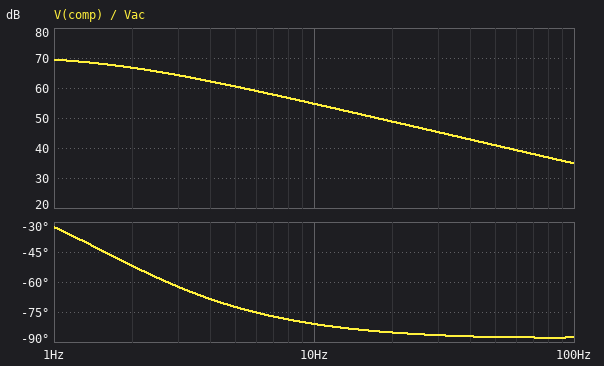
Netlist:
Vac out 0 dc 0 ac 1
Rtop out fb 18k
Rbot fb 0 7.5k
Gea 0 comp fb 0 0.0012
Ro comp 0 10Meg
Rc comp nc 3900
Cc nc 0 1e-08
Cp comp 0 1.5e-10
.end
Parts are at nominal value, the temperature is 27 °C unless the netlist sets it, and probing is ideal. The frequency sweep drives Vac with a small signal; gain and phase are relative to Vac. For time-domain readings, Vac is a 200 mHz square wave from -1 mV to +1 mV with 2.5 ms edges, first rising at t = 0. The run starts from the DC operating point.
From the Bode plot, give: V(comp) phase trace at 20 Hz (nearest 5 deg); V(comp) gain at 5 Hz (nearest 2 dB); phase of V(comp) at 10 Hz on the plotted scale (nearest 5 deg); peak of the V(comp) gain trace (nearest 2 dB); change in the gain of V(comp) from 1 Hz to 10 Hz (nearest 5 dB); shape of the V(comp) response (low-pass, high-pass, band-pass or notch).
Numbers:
-85 deg
60 dB
-80 deg
70 dB
-15 dB
low-pass
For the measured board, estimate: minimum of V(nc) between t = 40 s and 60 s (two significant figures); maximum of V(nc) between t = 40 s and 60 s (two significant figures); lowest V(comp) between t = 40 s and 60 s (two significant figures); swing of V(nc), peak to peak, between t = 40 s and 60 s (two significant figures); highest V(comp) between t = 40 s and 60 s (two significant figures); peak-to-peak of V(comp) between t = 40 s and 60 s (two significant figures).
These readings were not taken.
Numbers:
-3.5 V
3.5 V
-3.5 V
7.1 V
3.5 V
7.1 V
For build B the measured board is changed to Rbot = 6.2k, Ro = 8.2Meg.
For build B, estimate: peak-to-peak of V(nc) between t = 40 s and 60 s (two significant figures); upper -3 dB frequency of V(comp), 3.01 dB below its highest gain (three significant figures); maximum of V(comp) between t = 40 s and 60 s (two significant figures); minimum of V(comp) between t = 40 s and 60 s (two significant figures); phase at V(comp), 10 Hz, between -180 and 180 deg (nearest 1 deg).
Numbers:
5.0 V
1.91 Hz
2.5 V
-2.5 V
-79 deg
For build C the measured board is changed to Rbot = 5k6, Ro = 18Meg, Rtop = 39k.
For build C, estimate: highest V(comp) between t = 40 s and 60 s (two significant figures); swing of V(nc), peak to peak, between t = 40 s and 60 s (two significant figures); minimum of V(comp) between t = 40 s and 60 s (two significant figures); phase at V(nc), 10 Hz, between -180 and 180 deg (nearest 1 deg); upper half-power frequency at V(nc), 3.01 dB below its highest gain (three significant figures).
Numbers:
2.7 V
5.4 V
-2.7 V
-85 deg
871 mHz
